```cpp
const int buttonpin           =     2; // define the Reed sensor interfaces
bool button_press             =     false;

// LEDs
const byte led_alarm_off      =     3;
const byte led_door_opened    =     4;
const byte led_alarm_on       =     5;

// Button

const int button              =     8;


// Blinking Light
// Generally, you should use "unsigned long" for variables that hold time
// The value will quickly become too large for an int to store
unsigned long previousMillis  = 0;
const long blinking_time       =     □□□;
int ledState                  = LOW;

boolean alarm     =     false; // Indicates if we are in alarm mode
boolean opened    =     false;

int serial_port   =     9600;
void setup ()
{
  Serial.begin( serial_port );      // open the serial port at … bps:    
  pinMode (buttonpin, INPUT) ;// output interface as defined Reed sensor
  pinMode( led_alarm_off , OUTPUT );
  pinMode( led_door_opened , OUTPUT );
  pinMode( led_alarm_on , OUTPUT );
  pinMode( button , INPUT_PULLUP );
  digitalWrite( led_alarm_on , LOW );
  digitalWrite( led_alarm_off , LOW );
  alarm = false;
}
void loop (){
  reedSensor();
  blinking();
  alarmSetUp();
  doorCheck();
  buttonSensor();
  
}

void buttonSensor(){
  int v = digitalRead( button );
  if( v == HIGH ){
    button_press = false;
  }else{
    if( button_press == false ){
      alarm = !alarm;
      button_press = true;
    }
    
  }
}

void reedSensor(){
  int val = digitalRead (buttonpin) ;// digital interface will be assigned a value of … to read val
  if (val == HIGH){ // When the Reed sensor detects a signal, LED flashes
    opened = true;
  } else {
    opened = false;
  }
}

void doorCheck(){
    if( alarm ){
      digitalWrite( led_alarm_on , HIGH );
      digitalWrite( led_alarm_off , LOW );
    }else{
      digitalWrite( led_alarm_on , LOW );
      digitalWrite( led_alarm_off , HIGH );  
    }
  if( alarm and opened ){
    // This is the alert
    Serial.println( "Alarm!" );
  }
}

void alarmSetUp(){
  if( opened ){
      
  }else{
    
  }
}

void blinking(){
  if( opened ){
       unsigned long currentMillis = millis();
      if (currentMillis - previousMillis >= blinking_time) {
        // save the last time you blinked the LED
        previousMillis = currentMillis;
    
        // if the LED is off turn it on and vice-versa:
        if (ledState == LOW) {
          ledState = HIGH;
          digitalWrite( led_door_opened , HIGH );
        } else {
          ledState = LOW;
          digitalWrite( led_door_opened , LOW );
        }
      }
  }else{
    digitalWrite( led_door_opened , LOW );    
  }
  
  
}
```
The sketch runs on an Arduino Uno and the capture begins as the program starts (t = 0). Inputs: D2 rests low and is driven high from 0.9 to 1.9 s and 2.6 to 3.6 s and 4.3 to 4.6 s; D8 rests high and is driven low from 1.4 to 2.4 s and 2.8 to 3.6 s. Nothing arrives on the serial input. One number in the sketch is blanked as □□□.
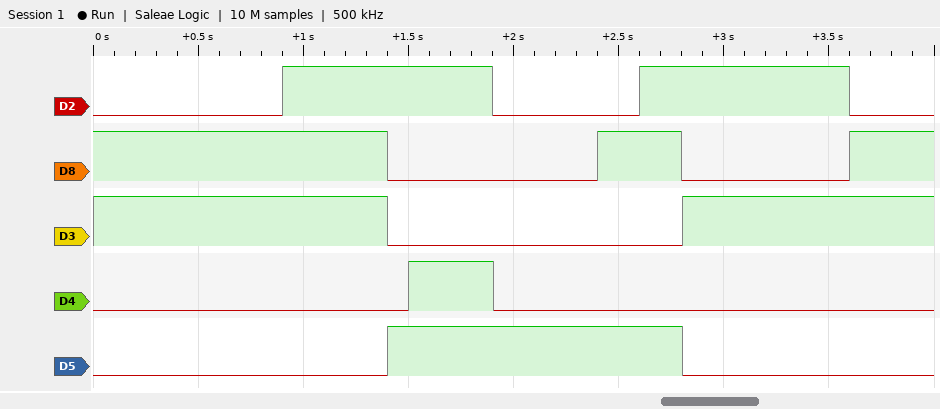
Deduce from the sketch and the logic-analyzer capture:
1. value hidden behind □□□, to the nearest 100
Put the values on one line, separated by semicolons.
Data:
1500
